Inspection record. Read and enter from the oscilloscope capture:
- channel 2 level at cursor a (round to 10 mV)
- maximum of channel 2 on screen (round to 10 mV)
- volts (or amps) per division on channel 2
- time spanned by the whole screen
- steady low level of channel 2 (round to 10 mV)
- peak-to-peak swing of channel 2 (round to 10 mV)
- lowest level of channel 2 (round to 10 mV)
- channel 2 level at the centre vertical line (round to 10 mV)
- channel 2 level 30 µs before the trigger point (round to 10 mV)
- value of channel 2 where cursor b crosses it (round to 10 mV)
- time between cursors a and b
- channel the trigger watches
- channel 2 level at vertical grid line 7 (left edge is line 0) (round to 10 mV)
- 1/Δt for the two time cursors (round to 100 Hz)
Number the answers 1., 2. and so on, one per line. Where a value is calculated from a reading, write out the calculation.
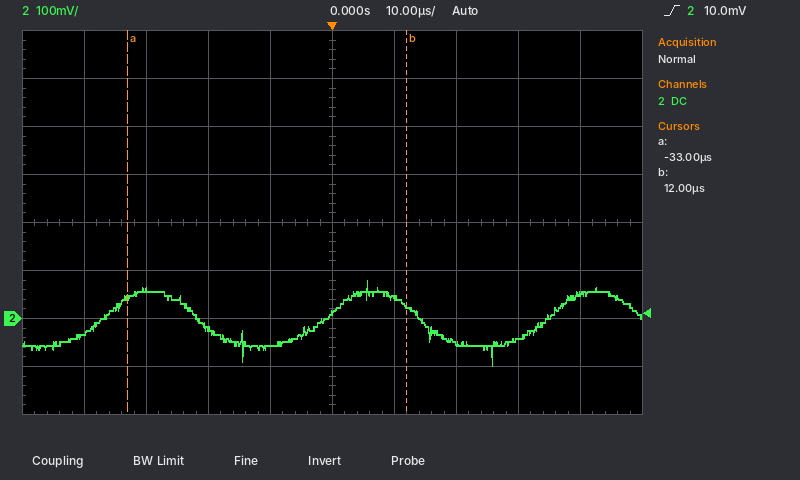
1. 40 mV
2. 80 mV
3. 100 mV
4. 100 µs
5. -60 mV
6. 80 mV − (-100 mV) = 180 mV
7. -100 mV
8. 10 mV
9. 60 mV
10. 30 mV
11. 12 µs − (-33 µs) = 45 µs
12. channel 2
13. -50 mV
14. 1 / 45 µs ≈ 22.2 kHz
